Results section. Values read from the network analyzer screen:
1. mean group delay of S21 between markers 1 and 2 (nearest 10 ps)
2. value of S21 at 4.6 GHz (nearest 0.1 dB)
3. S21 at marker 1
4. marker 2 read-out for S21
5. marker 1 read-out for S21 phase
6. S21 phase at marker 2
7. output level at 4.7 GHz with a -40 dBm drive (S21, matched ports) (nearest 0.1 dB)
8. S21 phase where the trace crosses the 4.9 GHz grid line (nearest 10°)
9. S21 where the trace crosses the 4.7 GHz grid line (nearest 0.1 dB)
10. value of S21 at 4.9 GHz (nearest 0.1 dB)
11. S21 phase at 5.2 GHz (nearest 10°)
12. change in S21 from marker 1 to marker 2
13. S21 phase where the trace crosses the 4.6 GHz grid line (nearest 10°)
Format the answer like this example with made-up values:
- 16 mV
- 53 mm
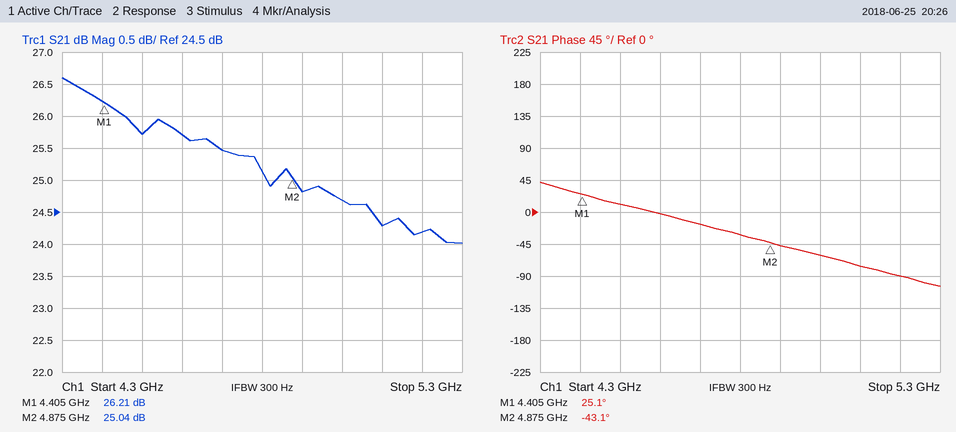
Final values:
- 400 ps
- 25.7 dB
- 26.21 dB
- 25.04 dB
- 25.1°
- -43.1°
- -14.5 dBm
- -50°
- 25.5 dB
- 24.8 dB
- -90°
- -1.17 dB
- 0°
